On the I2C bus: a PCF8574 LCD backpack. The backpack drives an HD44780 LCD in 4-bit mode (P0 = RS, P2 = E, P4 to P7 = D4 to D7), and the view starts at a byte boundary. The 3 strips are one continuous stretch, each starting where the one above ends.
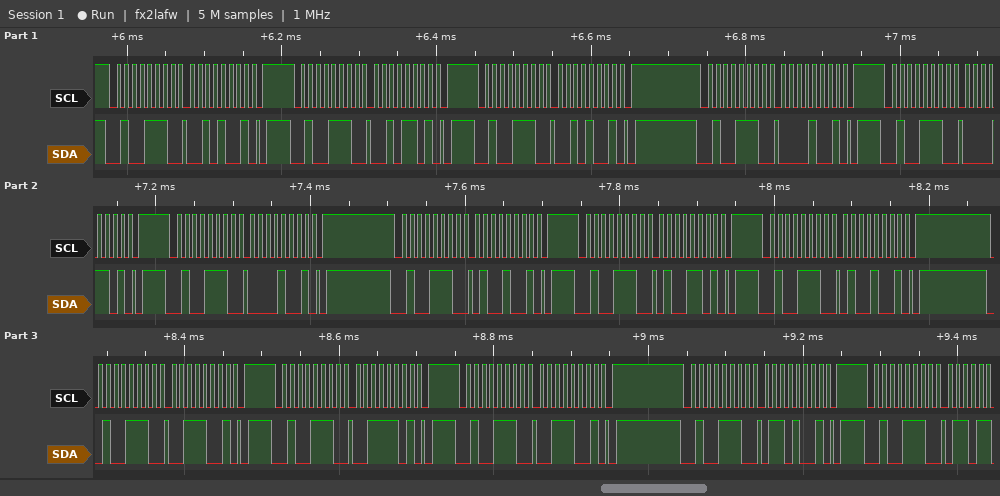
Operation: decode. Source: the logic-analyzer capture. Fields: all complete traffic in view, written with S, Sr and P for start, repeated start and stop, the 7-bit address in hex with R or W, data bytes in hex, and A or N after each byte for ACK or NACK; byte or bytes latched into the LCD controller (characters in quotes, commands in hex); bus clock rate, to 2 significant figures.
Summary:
S 27W A 29 A P S 27W A 2D A P S 27W A 29 A P S 27W A 09 A P S 27W A 0D A P S 27W A 09 A P S 27W A 49 A P S 27W A 4D A P S 27W A 49 A P S 27W A 39 A P S 27W A 3D A P S 27W A 39 A P S 27W A 69 A P S 27W A
' ' 'C'
100 kHz
